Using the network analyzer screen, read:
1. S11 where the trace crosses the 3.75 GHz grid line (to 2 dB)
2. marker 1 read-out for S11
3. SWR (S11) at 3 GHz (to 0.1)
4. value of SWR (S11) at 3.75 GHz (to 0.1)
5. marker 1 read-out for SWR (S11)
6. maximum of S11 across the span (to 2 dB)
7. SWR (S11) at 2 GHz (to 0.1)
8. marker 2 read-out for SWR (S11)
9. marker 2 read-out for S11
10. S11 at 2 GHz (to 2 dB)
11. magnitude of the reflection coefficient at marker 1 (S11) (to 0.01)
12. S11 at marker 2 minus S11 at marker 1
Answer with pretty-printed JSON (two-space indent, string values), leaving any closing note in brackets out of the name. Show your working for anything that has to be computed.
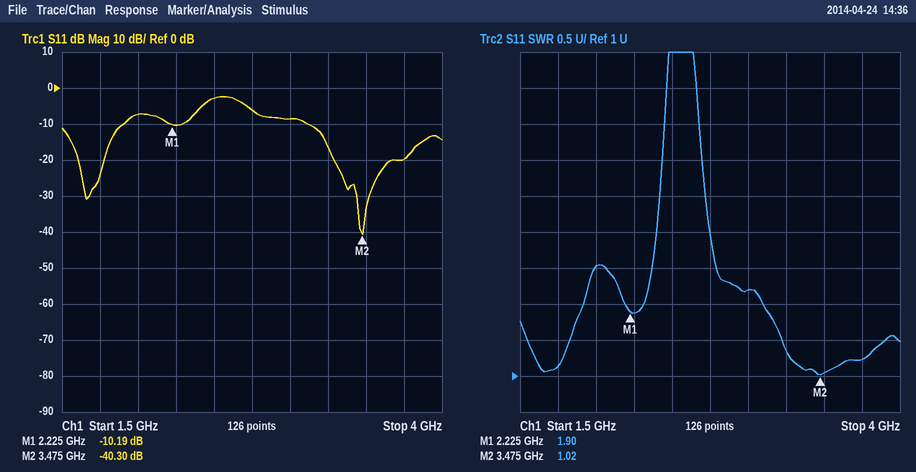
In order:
{
  "S11 where the trace crosses the 3.75 GHz grid line": "-20 dB",
  "marker 1 read-out for S11": "-10.19 dB",
  "SWR (S11) at 3 GHz": "2.2",
  "value of SWR (S11) at 3.75 GHz": "1.2",
  "marker 1 read-out for SWR": "1.90",
  "maximum of S11 across the span": "-2 dB",
  "SWR (S11) at 2 GHz": "2.5",
  "marker 2 read-out for SWR": "1.02",
  "marker 2 read-out for S11": "-40.30 dB",
  "S11 at 2 GHz": "-8 dB",
  "magnitude of the reflection coefficient at marker 1 (S11)": "10^(-10.19/20) ≈ 0.31",
  "S11 at marker 2 minus S11 at marker 1": "-40.3 − (-10.19) = -30.11 dB"
}
